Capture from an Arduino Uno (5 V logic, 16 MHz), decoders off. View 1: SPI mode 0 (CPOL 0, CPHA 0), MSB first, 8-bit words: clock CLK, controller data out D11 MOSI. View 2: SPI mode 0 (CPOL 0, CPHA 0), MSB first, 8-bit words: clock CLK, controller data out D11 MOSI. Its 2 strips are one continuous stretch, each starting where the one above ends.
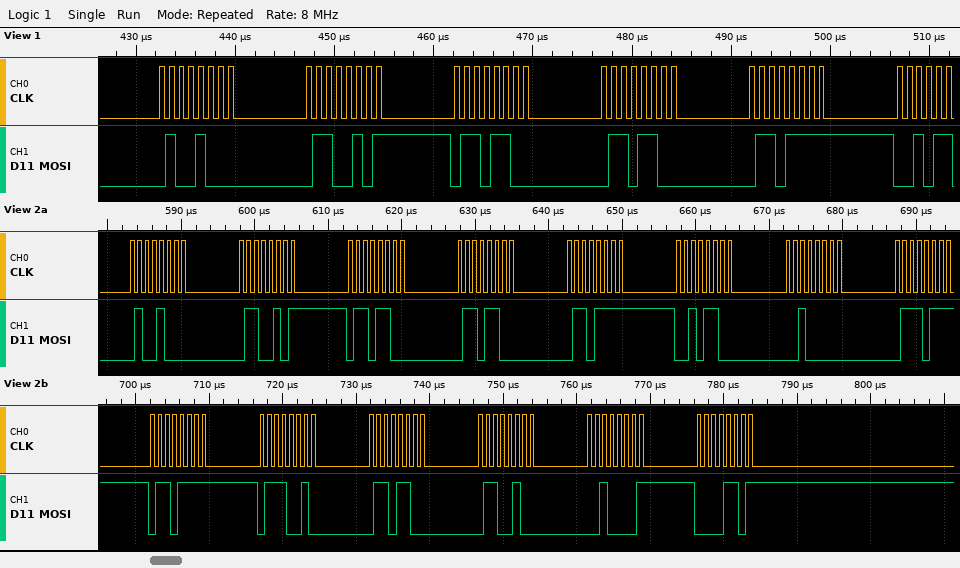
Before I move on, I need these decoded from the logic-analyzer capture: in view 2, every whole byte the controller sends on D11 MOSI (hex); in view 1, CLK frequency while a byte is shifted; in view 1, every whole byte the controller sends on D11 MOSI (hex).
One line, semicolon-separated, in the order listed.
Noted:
0x48 0x65 0x6C 0x6C 0x6F 0x2C 0x20 0x77 0x6F 0x72 0x6C 0x64 0x21 0x0D; 1 MHz; 48 65 6C 6C 6F
